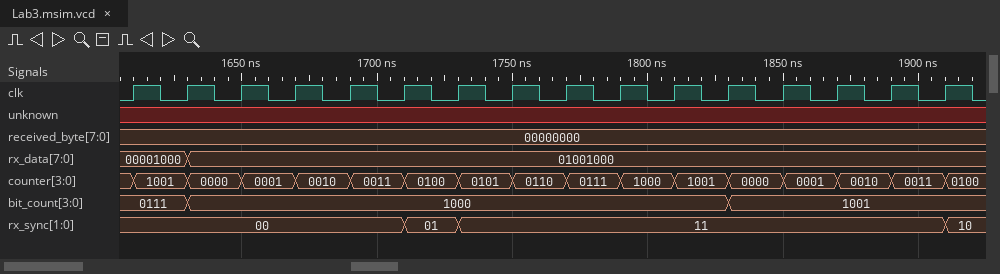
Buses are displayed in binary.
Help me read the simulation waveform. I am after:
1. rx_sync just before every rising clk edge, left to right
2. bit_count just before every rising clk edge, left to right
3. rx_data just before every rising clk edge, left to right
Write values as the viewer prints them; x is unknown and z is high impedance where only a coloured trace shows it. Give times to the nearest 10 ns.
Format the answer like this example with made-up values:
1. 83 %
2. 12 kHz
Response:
1. 00, 00, 00, 00, 00, 00, 01, 11, 11, 11, 11, 11, 11, 11, 11, 11
2. 0111, 0111, 1000, 1000, 1000, 1000, 1000, 1000, 1000, 1000, 1000, 1000, 1001, 1001, 1001, 1001
3. 00001000, 00001000, 01001000, 01001000, 01001000, 01001000, 01001000, 01001000, 01001000, 01001000, 01001000, 01001000, 01001000, 01001000, 01001000, 01001000
